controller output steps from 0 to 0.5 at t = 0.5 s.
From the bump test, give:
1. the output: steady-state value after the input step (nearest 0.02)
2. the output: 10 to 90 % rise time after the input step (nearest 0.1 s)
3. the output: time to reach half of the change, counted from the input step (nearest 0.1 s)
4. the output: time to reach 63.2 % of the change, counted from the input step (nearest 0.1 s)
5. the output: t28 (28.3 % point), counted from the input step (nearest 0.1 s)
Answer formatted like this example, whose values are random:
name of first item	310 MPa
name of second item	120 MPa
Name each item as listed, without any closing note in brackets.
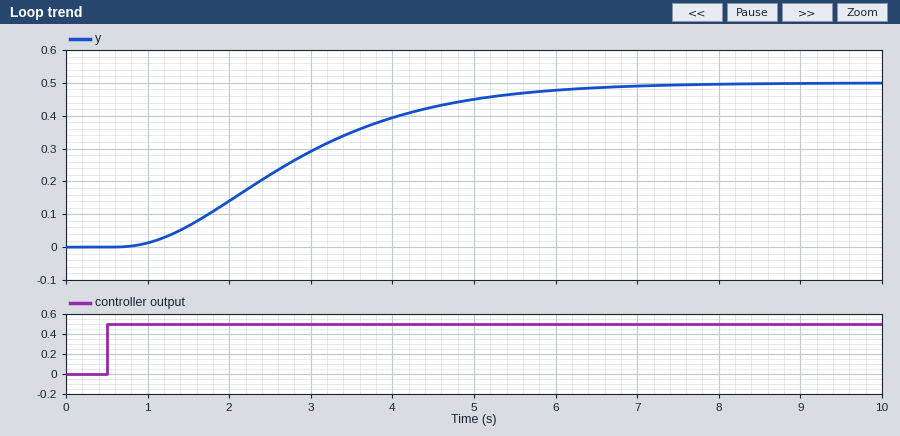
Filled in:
the output: steady-state value after the input step	0.50
the output: 10 to 90 % rise time after the input step	3.6 s
the output: time to reach half of the change, counted from the input step	2.2 s
the output: time to reach 63.2 % of the change, counted from the input step	2.7 s
the output: t28 (28.3 % point), counted from the input step	1.5 s
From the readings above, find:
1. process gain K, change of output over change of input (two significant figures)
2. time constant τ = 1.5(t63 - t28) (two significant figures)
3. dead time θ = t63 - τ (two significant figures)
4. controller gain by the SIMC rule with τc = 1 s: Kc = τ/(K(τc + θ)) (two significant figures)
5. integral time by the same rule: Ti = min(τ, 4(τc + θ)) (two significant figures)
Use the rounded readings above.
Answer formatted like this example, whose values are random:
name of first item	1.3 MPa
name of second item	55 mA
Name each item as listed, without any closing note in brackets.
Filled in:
process gain K, change of output over change of input	1.0
time constant τ = 1.5(t63 - t28)	1.8 s
dead time θ = t63 - τ	0.90 s
controller gain by the SIMC rule with τc = 1 s: Kc = τ/(K(τc + θ))	0.95
integral time by the same rule: Ti = min(τ, 4(τc + θ))	1.8 s
